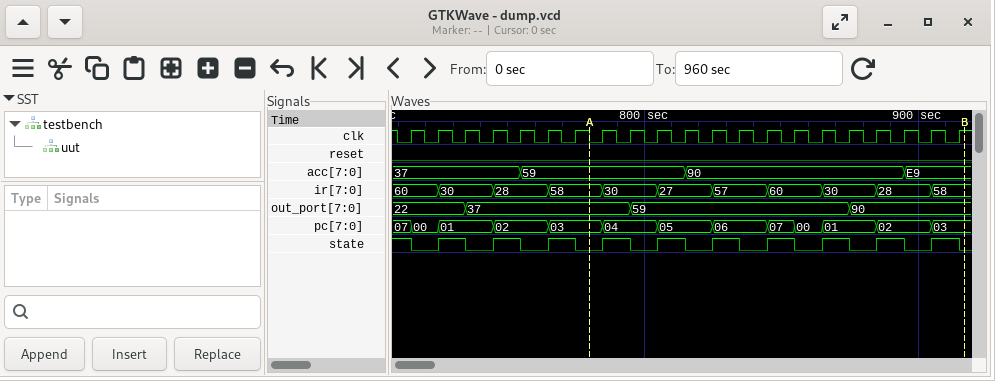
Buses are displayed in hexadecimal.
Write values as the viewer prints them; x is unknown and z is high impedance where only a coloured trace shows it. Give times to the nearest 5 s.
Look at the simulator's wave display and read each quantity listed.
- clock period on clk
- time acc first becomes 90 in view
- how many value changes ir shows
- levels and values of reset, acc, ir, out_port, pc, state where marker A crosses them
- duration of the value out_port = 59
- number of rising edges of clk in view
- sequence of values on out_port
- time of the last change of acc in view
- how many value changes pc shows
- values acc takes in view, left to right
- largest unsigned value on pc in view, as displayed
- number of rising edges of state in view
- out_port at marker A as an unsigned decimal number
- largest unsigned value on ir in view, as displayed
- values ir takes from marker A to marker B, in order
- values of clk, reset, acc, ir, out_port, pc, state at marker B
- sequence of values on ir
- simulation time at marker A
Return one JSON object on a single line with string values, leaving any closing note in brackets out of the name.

{"clock period on clk": "10 s", "time acc first becomes 90 in view": "815 s", "how many value changes ir shows": "10", "levels and values of reset, acc, ir, out_port, pc, state where marker A crosses them": "reset=0, acc=59, ir=58, out_port=37, pc=03, state=0", "duration of the value out_port = 59": "80 s", "number of rising edges of clk in view": "21", "sequence of values on out_port": "22, 37, 59, 90", "time of the last change of acc in view": "895 s", "how many value changes pc shows": "12", "values acc takes in view, left to right": "37, 59, 90, E9", "largest unsigned value on pc in view, as displayed": "07", "number of rising edges of state in view": "10", "out_port at marker A as an unsigned decimal number": "55", "largest unsigned value on ir in view, as displayed": "60", "values ir takes from marker A to marker B, in order": "58, 30, 27, 57, 60, 30, 28, 58", "values of clk, reset, acc, ir, out_port, pc, state at marker B": "clk=1, reset=0, acc=E9, ir=58, out_port=90, pc=03, state=0", "sequence of values on ir": "60, 30, 28, 58, 30, 27, 57, 60, 30, 28, 58", "simulation time at marker A": "780 s"}
